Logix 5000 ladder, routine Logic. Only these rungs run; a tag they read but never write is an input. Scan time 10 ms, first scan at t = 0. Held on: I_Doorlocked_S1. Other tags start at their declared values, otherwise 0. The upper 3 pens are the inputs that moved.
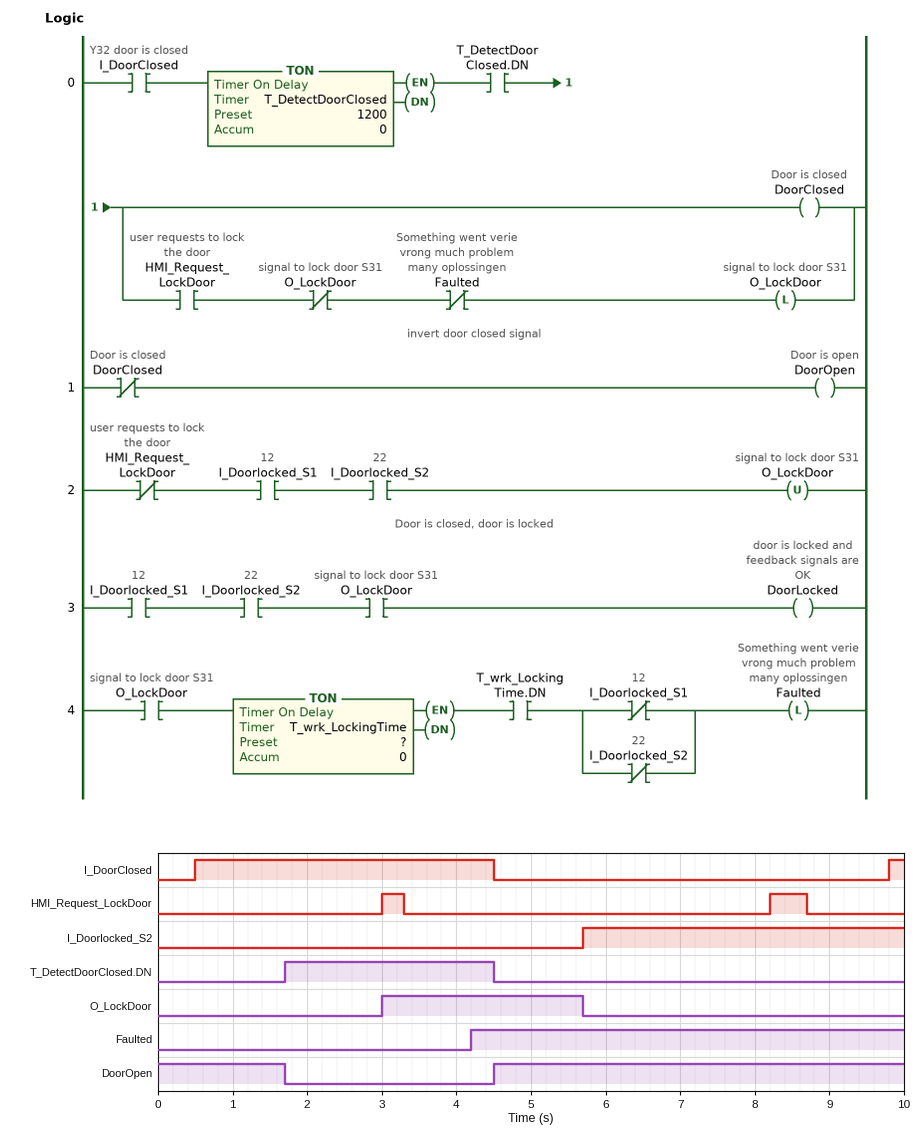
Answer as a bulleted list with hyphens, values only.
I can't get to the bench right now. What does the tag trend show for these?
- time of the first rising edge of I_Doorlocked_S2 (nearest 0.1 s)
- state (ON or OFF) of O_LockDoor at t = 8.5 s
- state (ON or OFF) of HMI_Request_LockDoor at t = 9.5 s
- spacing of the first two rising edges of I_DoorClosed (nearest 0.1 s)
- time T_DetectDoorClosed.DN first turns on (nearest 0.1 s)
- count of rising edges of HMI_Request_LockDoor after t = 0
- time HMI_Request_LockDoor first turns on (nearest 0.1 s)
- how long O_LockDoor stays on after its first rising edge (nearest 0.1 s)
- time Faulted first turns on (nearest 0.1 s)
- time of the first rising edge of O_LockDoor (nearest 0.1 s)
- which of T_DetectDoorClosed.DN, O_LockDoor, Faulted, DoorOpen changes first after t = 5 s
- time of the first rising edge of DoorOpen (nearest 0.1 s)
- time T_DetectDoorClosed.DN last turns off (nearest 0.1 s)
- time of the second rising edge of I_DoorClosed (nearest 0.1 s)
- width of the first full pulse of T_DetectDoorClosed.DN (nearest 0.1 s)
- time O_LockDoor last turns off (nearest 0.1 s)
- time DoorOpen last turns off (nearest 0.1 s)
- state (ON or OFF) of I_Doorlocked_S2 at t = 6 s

- 5.7 s
- OFF
- OFF
- 9.3 s
- 1.7 s
- 2
- 3.0 s
- 2.7 s
- 4.2 s
- 3.0 s
- O_LockDoor
- 4.5 s
- 4.5 s
- 9.8 s
- 2.8 s
- 5.7 s
- 1.7 s
- ON
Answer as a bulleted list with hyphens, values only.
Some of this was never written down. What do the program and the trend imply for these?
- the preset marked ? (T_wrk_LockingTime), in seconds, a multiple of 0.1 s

- 1.2 s
